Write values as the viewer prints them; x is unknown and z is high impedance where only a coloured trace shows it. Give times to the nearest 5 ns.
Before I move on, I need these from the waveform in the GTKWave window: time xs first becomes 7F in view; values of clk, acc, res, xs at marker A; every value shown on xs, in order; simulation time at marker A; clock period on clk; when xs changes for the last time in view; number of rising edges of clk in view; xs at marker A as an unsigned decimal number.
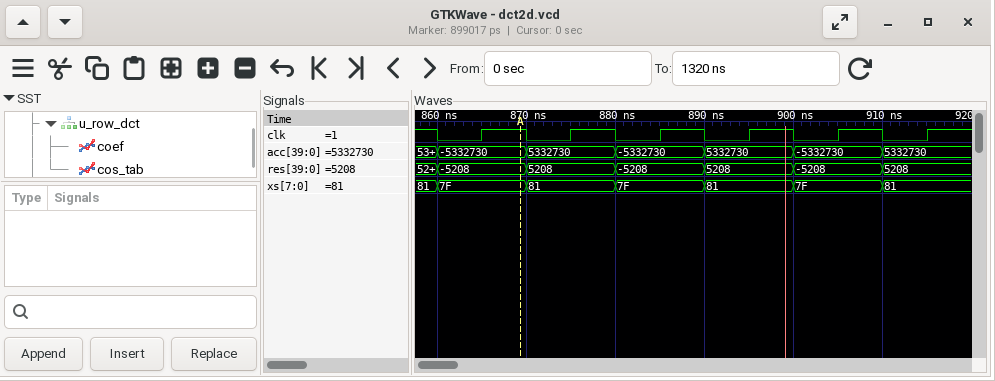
860 ns
clk=1, acc=-5332730, res=-5208, xs=7F
81, 7F, 81, 7F, 81, 7F, 81
870 ns
10 ns
910 ns
6
127
